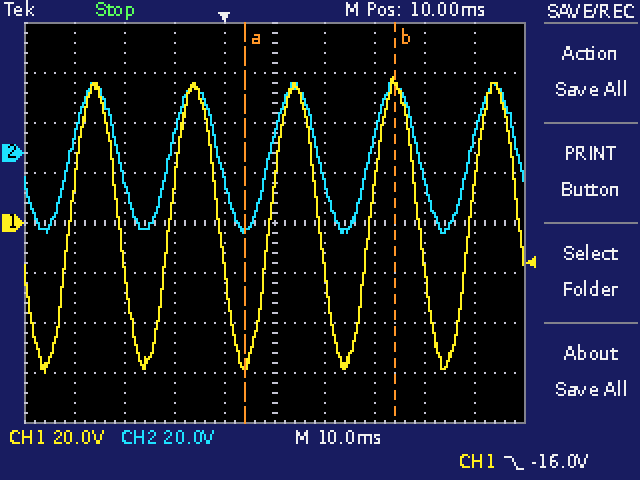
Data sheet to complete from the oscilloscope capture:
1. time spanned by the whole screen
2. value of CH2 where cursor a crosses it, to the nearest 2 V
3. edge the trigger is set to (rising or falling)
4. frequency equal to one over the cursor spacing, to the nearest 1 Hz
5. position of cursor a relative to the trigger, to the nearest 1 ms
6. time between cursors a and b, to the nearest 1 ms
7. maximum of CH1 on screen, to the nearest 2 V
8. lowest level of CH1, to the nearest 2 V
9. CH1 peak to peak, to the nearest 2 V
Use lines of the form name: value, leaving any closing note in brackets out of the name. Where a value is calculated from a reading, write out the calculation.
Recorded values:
time spanned by the whole screen: 100 ms
value of CH2 where cursor a crosses it, to the nearest 2 V: -30 V
edge the trigger is set to: falling
frequency equal to one over the cursor spacing, to the nearest 1 Hz: 1 / 30 ms ≈ 33 Hz
position of cursor a relative to the trigger, to the nearest 1 ms: +4 ms
time between cursors a and b, to the nearest 1 ms: 30 ms
maximum of CH1 on screen, to the nearest 2 V: 58 V
lowest level of CH1, to the nearest 2 V: -60 V
CH1 peak to peak, to the nearest 2 V: 58 V − (-60 V) = 118 V
